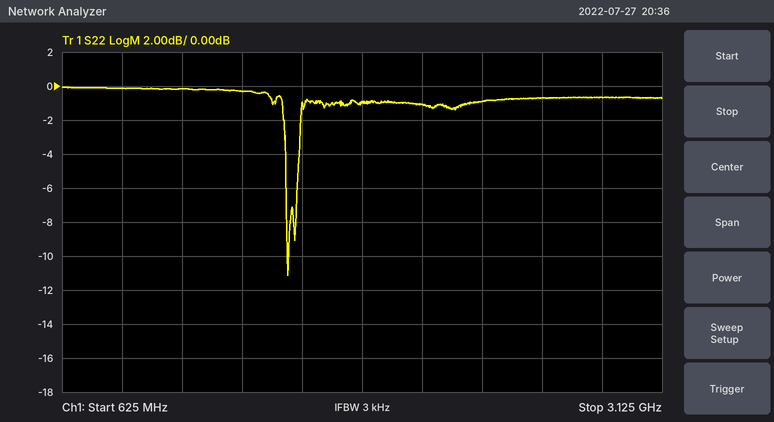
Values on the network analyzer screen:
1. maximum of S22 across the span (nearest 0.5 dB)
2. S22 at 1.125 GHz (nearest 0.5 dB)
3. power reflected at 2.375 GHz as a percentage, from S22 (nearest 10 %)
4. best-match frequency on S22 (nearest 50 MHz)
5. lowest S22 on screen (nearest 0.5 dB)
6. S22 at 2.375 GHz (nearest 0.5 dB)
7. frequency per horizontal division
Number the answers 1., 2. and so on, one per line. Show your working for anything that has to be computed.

1. 0.0 dB
2. 0.0 dB
3. 10^(-1/10) ≈ 79.4 %, so 80 % to the nearest 10 %
4. 1.55 GHz
5. -11.0 dB
6. -1.0 dB
7. 250 MHz
